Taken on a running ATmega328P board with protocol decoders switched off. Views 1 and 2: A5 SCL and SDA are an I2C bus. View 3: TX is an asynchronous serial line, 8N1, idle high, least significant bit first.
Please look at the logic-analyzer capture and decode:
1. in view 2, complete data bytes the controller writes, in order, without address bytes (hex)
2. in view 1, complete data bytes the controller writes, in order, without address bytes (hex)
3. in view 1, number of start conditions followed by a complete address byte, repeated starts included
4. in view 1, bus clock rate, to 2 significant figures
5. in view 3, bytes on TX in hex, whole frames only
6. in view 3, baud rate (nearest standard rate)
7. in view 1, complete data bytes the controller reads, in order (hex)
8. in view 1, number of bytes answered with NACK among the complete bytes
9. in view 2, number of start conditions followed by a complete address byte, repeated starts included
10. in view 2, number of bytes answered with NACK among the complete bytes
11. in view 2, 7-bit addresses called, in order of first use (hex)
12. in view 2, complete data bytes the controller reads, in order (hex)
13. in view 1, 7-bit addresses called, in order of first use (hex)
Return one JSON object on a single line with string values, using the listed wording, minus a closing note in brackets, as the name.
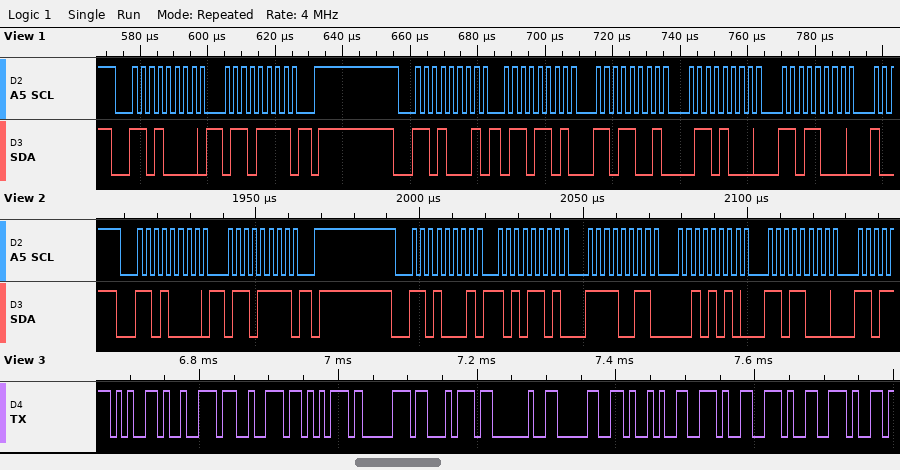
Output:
{"in view 2, complete data bytes the controller writes, in order, without address bytes": "6F", "in view 1, complete data bytes the controller writes, in order, without address bytes": "6F", "in view 1, number of start conditions followed by a complete address byte, repeated starts included": "2", "in view 1, bus clock rate, to 2 significant figures": "400 kHz", "in view 3, bytes on TX in hex, whole frames only": "65 72 72 75 70 74 20 30 29 2E 2E 2E", "in view 3, baud rate": "115200 baud", "in view 1, complete data bytes the controller reads, in order": "6D D9 68 D8", "in view 1, number of bytes answered with NACK among the complete bytes": "0", "in view 2, number of start conditions followed by a complete address byte, repeated starts included": "2", "in view 2, number of bytes answered with NACK among the complete bytes": "0", "in view 2, 7-bit addresses called, in order of first use": "0x68", "in view 2, complete data bytes the controller reads, in order": "AD F3 2A D8", "in view 1, 7-bit addresses called, in order of first use": "0x68"}
